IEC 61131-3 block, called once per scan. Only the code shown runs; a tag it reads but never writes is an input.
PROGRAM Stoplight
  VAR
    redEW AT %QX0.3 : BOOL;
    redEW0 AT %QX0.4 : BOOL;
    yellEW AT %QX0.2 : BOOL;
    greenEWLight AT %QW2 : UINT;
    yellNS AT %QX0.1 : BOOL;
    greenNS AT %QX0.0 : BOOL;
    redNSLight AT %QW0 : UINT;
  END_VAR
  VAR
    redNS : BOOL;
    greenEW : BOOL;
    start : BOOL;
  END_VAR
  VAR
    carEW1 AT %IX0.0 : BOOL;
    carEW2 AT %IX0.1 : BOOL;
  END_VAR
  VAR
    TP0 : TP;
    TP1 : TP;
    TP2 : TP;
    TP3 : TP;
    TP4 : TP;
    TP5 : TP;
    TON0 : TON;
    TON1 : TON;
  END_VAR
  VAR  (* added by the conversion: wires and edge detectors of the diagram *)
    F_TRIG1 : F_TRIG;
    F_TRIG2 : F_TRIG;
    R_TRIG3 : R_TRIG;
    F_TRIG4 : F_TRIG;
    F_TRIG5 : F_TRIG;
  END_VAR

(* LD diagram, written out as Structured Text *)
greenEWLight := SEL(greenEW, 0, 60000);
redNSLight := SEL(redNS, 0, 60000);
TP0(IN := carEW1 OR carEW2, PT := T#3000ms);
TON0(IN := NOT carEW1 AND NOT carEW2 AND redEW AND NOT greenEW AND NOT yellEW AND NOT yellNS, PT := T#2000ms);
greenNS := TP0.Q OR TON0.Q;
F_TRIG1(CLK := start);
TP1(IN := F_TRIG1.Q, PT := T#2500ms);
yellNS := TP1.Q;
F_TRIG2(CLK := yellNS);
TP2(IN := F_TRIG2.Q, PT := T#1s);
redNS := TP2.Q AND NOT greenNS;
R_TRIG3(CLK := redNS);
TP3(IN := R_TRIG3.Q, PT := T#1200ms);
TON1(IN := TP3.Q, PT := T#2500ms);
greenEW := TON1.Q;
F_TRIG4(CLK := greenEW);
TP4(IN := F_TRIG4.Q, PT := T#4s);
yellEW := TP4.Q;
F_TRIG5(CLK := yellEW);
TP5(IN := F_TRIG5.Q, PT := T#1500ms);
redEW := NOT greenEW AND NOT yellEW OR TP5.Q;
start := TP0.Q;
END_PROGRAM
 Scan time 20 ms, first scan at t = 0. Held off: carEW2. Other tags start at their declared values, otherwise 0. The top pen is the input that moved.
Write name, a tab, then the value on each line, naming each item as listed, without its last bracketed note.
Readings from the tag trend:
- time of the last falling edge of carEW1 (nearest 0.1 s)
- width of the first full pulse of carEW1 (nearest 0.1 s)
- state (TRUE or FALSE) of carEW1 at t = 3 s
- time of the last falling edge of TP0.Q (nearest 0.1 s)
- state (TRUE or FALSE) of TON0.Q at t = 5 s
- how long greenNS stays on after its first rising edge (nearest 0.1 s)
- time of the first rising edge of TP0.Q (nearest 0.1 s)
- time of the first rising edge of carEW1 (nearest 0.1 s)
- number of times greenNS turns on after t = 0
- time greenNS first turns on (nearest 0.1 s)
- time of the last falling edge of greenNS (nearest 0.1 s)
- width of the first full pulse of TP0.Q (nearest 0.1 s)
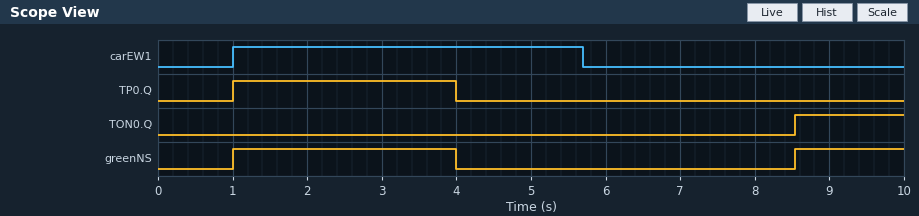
time of the last falling edge of carEW1	5.7 s
width of the first full pulse of carEW1	4.7 s
state (TRUE or FALSE) of carEW1 at t = 3 s	TRUE
time of the last falling edge of TP0.Q	4.0 s
state (TRUE or FALSE) of TON0.Q at t = 5 s	FALSE
how long greenNS stays on after its first rising edge	3.0 s
time of the first rising edge of TP0.Q	1.0 s
time of the first rising edge of carEW1	1.0 s
number of times greenNS turns on after t = 0	2
time greenNS first turns on	1.0 s
time of the last falling edge of greenNS	4.0 s
width of the first full pulse of TP0.Q	3.0 s
